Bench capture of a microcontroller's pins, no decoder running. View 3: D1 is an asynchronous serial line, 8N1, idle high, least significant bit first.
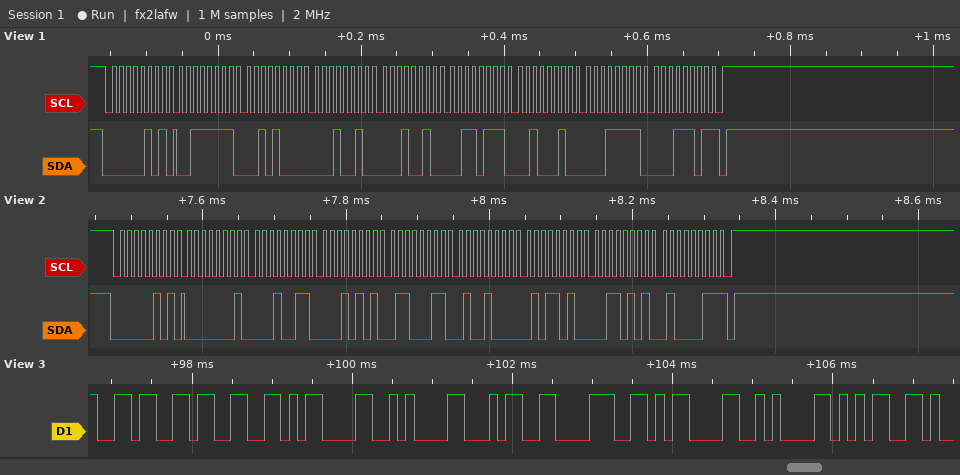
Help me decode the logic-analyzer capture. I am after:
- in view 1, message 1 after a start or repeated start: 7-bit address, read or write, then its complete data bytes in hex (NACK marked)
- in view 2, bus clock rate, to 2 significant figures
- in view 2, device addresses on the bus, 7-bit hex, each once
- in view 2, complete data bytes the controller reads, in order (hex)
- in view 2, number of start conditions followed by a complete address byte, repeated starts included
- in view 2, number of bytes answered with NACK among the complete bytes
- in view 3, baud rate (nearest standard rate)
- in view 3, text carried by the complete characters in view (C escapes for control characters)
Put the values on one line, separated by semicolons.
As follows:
0x02 read: 3F 28 12 12 37 22 1F 1D NACK; 100 kHz; 0x02; 01 13 15 63 48 5A 35 43; 1; 1; 9600 baud; "63\r\n48\r\n5"
